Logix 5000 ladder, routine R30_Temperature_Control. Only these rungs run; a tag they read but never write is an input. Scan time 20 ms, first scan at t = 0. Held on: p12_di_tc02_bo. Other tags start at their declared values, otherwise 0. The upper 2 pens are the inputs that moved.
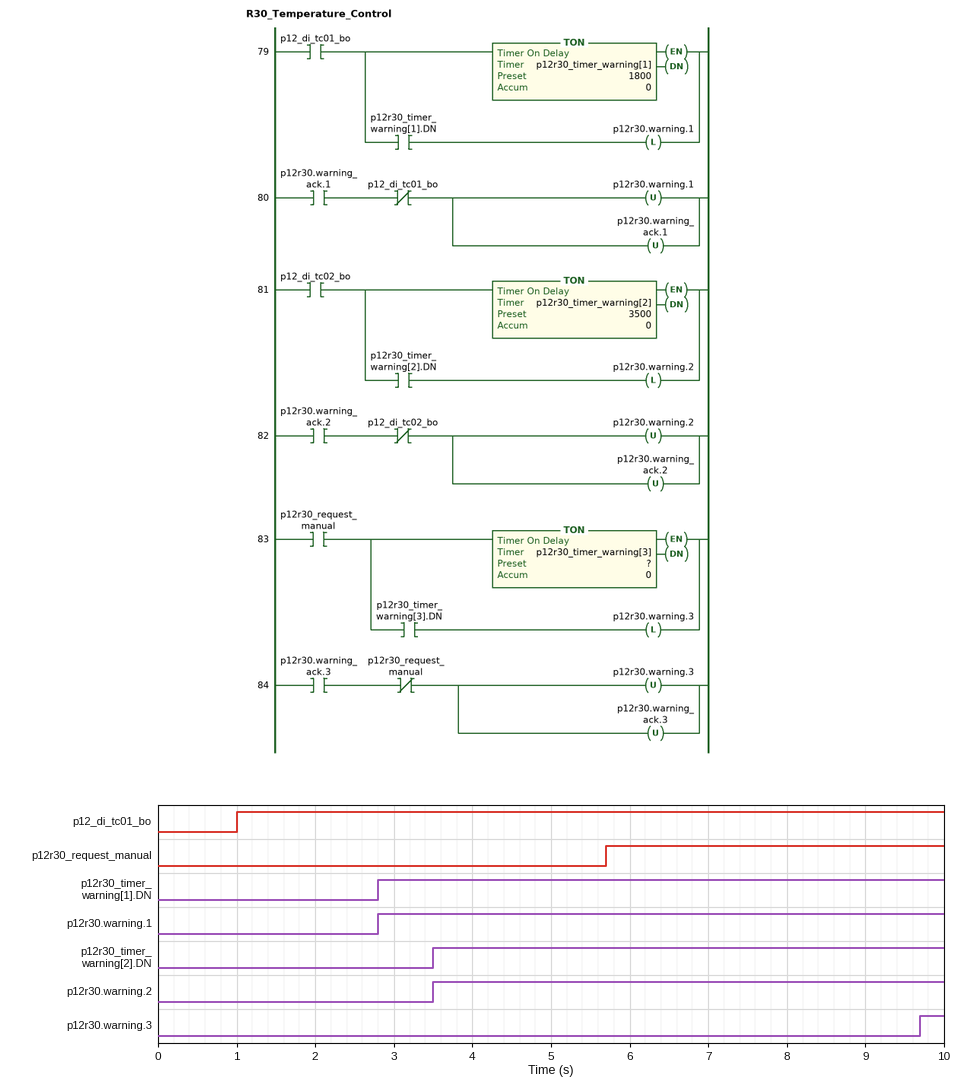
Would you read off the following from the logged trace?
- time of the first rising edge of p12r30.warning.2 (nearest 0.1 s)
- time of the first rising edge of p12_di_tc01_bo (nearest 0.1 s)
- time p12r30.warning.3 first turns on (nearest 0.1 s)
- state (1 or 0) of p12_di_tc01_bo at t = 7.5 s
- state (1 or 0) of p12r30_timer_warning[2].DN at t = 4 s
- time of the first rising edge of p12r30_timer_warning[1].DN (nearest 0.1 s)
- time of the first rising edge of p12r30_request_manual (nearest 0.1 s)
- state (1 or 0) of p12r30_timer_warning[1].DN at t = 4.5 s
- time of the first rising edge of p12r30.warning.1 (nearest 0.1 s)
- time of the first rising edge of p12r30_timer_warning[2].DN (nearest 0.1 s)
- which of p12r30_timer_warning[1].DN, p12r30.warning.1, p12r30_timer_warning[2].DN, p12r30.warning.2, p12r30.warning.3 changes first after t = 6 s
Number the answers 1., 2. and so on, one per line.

1. 3.5 s
2. 1.0 s
3. 9.7 s
4. 1
5. 1
6. 2.8 s
7. 5.7 s
8. 1
9. 2.8 s
10. 3.5 s
11. p12r30.warning.3
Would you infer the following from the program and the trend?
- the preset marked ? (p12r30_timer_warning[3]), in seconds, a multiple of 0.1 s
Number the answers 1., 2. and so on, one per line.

1. 4.0 s
